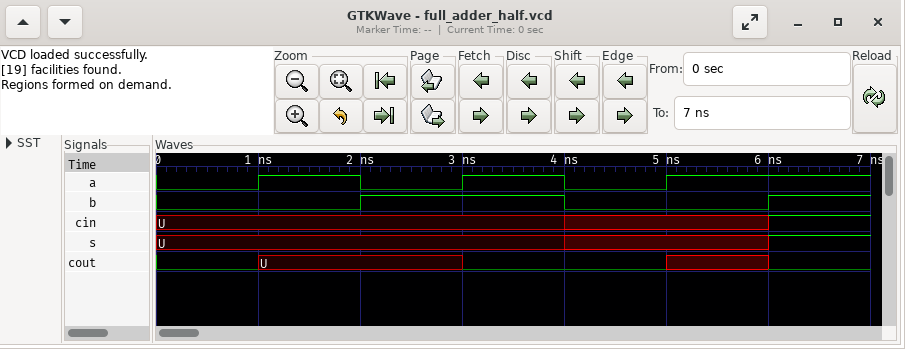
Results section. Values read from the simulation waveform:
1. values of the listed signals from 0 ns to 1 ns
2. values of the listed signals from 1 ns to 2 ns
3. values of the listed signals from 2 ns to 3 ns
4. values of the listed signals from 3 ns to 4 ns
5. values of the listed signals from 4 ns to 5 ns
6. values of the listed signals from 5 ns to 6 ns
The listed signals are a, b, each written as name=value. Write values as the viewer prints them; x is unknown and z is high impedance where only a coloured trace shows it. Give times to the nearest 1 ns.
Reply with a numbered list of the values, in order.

1. a=0, b=0
2. a=1, b=0
3. a=0, b=1
4. a=1, b=1
5. a=0, b=0
6. a=1, b=0
